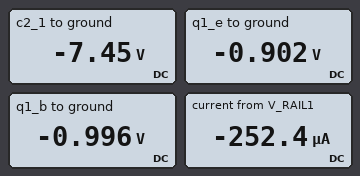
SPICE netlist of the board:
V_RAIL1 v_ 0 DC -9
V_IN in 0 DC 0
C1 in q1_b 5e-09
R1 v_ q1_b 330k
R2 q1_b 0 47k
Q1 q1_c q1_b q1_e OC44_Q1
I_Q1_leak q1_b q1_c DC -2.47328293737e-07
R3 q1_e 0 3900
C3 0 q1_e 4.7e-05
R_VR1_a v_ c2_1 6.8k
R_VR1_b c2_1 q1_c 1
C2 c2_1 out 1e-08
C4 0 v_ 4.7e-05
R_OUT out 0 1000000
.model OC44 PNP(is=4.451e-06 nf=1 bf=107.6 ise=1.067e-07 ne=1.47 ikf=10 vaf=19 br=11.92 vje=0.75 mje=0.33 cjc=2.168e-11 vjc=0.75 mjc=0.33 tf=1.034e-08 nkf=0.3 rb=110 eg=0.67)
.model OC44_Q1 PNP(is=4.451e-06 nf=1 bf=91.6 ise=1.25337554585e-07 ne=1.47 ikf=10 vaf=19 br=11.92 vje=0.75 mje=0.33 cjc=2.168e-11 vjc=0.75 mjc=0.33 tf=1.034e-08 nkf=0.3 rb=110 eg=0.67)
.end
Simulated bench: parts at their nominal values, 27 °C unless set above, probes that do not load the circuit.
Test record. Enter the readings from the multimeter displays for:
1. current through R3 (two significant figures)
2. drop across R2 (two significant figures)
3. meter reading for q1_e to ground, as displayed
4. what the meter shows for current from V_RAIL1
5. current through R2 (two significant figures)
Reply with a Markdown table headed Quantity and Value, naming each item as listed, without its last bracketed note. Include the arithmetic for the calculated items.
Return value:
| Quantity | Value |
|---|---|
| current through R3 | (0 V - (-902 mV)) / 3.9 kΩ = 230 µA |
| drop across R2 | 0 V - (-996 mV) = 1.0 V |
| meter reading for q1_e to ground, as displayed | -0.902 V |
| what the meter shows for current from V_RAIL1 | -252.4 µA |
| current through R2 | (0 V - (-996 mV)) / 47 kΩ = 21 µA |
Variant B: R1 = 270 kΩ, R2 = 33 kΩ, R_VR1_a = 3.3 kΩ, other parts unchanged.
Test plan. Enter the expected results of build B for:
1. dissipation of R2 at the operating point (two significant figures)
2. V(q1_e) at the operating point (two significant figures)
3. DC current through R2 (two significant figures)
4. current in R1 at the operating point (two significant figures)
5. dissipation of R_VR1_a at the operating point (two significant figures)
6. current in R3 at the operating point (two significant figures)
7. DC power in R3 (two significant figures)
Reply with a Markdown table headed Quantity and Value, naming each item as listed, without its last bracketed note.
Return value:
| Quantity | Value |
|---|---|
| dissipation of R2 at the operating point | 25 µW |
| V(q1_e) at the operating point | -810 mV |
| DC current through R2 | 27 µA |
| current in R1 at the operating point | 30 µA |
| dissipation of R_VR1_a at the operating point | 140 µW |
| current in R3 at the operating point | 210 µA |
| DC power in R3 | 170 µW |
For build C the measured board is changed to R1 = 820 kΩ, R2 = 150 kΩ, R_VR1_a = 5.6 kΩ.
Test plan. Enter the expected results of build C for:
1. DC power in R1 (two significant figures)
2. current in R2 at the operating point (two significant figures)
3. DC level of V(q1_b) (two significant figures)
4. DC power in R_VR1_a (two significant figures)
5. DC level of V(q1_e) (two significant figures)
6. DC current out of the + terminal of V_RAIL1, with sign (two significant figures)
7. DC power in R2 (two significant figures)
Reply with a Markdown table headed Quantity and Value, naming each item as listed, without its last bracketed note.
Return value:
| Quantity | Value |
|---|---|
| DC power in R1 | 78 µW |
| current in R2 at the operating point | 6.7 µA |
| DC level of V(q1_b) | -1.0 V |
| DC power in R_VR1_a | 300 µW |
| DC level of V(q1_e) | -910 mV |
| DC current out of the + terminal of V_RAIL1, with sign | -240 µA |
| DC power in R2 | 6.7 µW |
